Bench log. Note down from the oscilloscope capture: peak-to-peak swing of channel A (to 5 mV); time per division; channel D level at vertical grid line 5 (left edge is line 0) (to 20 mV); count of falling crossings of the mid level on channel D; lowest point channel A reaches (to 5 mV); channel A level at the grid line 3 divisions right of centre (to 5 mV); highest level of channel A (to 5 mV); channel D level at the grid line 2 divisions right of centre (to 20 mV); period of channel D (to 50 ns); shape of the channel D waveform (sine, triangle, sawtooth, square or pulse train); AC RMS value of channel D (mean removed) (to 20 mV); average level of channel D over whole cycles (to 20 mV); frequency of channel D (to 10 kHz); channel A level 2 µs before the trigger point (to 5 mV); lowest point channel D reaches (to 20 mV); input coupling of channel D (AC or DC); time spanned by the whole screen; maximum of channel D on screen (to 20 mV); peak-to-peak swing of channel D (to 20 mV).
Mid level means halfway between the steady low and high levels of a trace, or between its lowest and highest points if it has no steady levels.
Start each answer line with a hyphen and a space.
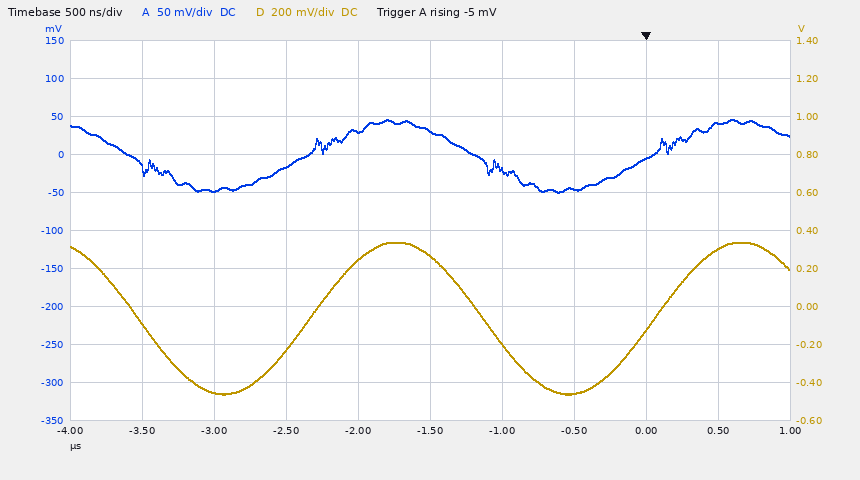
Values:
- 95 mV
- 500 ns
- 260 mV
- 2
- -50 mV
- -5 mV
- 45 mV
- -460 mV
- 2.40 µs
- sine
- 280 mV
- -60 mV
- 420 kHz
- 30 mV
- -460 mV
- DC
- 5 µs
- 340 mV
- 800 mV
